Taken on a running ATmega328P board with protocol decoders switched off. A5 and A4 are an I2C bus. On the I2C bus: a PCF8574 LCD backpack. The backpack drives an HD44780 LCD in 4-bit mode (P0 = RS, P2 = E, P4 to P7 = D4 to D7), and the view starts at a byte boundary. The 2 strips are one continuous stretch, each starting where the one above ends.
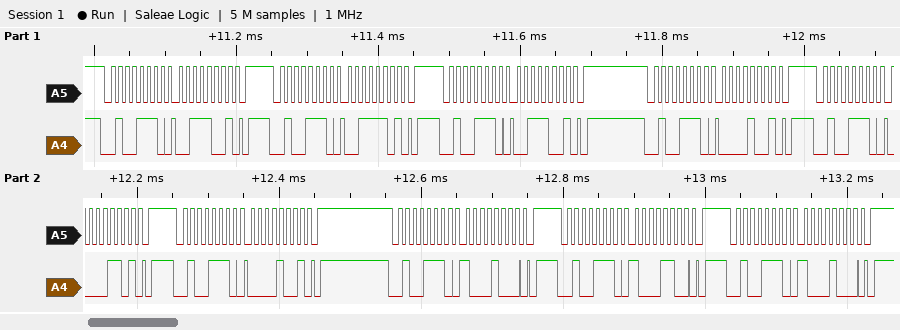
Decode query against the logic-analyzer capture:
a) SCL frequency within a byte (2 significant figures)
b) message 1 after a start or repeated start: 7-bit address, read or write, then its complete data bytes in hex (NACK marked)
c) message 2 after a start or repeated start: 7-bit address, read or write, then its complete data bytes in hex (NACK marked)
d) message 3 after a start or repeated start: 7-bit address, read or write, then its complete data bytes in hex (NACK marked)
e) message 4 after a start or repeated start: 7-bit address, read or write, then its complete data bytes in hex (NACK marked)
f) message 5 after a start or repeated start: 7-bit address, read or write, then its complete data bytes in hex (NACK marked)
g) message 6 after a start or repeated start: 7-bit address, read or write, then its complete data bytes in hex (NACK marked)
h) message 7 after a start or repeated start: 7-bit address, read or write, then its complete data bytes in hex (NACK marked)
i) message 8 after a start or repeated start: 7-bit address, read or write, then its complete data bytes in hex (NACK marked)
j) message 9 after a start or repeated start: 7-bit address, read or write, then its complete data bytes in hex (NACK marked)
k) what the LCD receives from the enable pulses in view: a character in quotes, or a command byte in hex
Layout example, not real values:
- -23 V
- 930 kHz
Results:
- 100 kHz
- 0x27 write: 39
- 0x27 write: 3D
- 0x27 write: 39
- 0x27 write: 09
- 0x27 write: 0D
- 0x27 write: 09
- 0x27 write: 88
- 0x27 write: 8C
- 0x27 write: 88
- '0'
